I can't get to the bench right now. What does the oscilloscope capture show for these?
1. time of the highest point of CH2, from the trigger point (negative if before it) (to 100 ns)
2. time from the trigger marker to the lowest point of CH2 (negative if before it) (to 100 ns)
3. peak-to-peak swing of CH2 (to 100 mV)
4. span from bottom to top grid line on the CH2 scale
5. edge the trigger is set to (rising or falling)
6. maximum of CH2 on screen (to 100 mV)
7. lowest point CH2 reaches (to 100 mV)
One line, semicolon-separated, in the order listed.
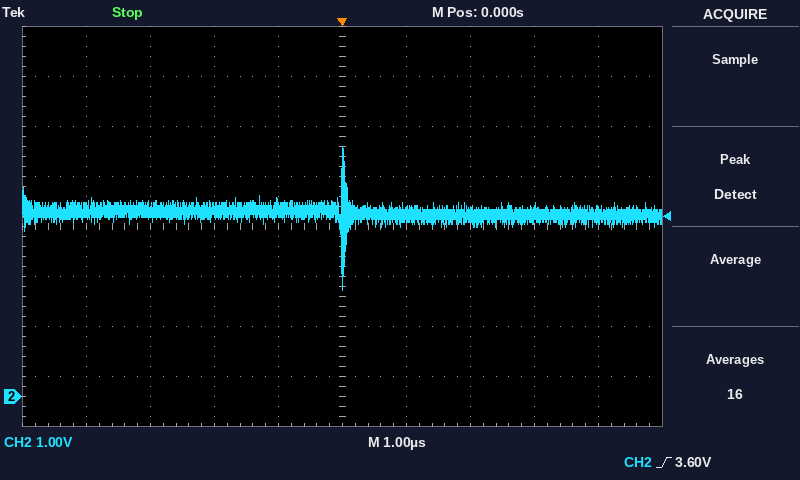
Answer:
0.0 µs; 0.0 µs; 2.9 V; 8 V; rising; 5.0 V; 2.1 V
